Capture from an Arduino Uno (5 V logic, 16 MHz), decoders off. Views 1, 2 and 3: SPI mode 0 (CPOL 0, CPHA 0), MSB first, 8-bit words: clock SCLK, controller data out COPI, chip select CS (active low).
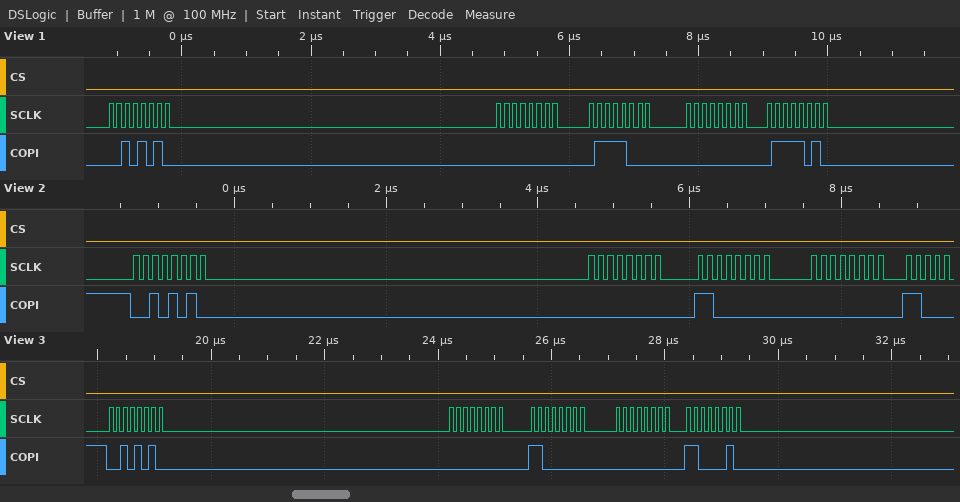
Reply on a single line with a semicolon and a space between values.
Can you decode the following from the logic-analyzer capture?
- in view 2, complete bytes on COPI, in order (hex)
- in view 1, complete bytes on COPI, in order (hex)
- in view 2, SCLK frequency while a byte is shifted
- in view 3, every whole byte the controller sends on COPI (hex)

2A 00 C0 00; 2A 00 78 00 7A; 8 MHz; 2A 00 C0 00 C2
